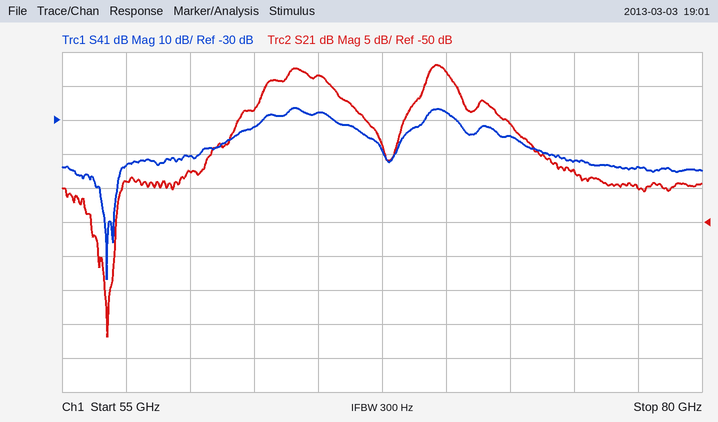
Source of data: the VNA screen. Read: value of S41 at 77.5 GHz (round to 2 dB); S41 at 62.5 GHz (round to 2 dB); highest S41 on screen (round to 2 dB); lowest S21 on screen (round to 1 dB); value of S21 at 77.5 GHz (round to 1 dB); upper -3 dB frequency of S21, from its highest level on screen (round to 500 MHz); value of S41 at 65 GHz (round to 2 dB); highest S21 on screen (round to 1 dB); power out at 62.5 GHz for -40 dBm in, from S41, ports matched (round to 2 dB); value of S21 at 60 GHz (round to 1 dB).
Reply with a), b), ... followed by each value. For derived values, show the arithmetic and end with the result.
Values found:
a) -44 dB
b) -32 dB
c) -26 dB
d) -67 dB
e) -45 dB
f) 70.5 GHz
g) -28 dB
h) -27 dB
i) -40 dBm + (-32 dB) = -72 dBm
j) -43 dB
